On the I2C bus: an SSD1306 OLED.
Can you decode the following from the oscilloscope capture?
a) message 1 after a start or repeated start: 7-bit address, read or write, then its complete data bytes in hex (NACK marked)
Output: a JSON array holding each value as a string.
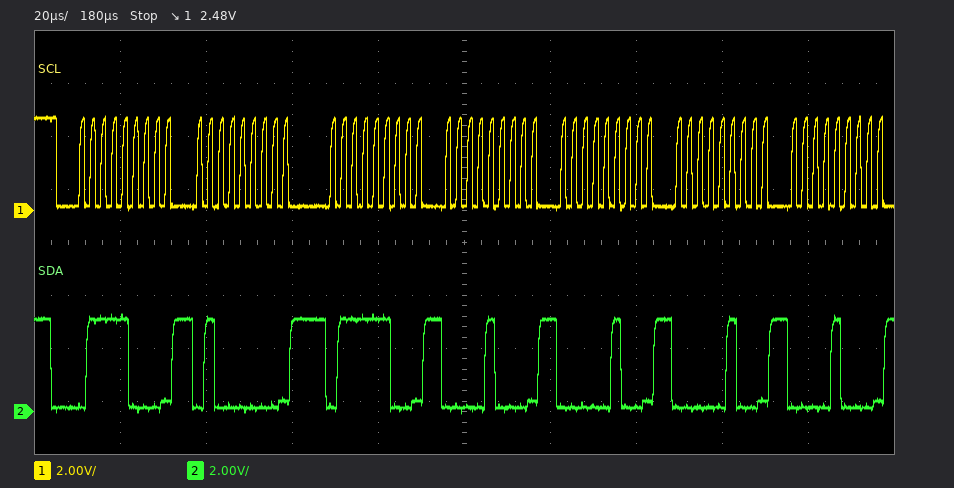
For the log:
["0x3C write: 40 7C 08 04 04 08"]
